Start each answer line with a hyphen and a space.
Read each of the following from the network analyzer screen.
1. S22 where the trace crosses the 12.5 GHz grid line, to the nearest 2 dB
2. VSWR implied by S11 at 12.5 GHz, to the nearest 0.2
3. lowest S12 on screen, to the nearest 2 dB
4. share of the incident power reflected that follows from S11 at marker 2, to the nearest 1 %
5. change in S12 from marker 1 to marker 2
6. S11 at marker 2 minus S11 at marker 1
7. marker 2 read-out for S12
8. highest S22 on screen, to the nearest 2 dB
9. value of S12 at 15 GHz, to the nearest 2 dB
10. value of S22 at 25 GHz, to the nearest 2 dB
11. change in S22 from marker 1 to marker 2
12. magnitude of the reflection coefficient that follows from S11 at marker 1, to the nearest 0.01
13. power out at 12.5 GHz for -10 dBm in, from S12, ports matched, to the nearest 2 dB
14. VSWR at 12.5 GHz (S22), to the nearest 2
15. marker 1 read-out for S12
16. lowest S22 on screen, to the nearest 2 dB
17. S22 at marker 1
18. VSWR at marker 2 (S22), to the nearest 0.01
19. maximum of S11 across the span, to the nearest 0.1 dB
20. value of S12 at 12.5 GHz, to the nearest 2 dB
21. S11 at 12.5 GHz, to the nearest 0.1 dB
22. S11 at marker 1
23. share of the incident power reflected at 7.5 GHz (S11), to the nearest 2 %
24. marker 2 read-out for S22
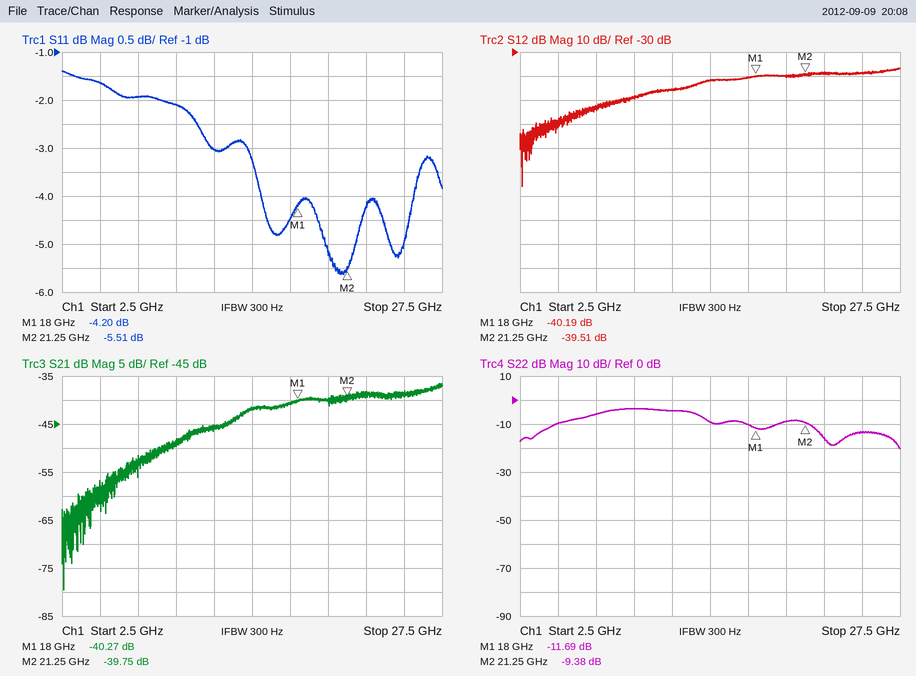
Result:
- -4 dB
- 5.8
- -86 dB
- 28 %
- 0.68 dB
- -1.31 dB
- -39.51 dB
- -4 dB
- -42 dB
- -14 dB
- 2.31 dB
- 0.62
- -56 dBm
- 4
- -40.19 dB
- -20 dB
- -11.69 dB
- 2.03
- -1.4 dB
- -46 dB
- -3.0 dB
- -4.20 dB
- 64 %
- -9.38 dB
